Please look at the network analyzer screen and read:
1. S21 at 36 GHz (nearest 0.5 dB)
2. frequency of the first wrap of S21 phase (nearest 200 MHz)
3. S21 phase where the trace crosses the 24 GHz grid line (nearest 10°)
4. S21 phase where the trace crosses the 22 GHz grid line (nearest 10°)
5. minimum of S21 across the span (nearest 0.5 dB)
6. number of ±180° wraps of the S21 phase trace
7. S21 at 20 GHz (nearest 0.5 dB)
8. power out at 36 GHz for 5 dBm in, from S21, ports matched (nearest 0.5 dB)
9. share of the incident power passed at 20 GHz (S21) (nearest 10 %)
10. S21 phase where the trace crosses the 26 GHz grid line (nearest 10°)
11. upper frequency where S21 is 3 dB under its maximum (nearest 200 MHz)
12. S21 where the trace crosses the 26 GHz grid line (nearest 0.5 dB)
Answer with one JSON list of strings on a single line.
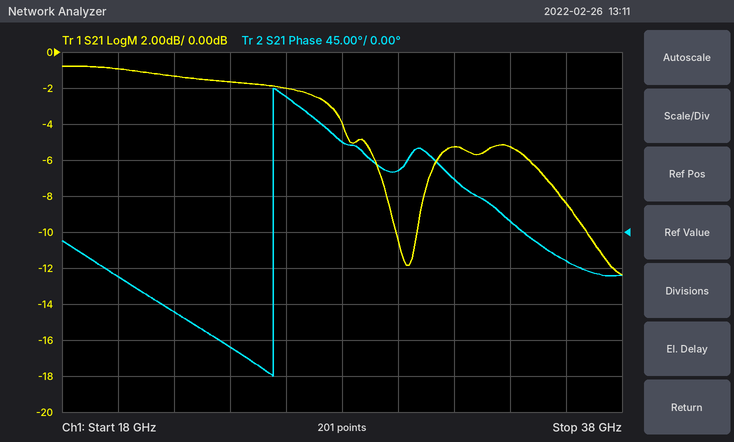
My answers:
["-8.5 dB", "25.6 GHz", "-140°", "-100°", "-12.5 dB", "1", "-1.0 dB", "-3.5 dBm", "80 %", "170°", "28.0 GHz", "-2.0 dB"]
